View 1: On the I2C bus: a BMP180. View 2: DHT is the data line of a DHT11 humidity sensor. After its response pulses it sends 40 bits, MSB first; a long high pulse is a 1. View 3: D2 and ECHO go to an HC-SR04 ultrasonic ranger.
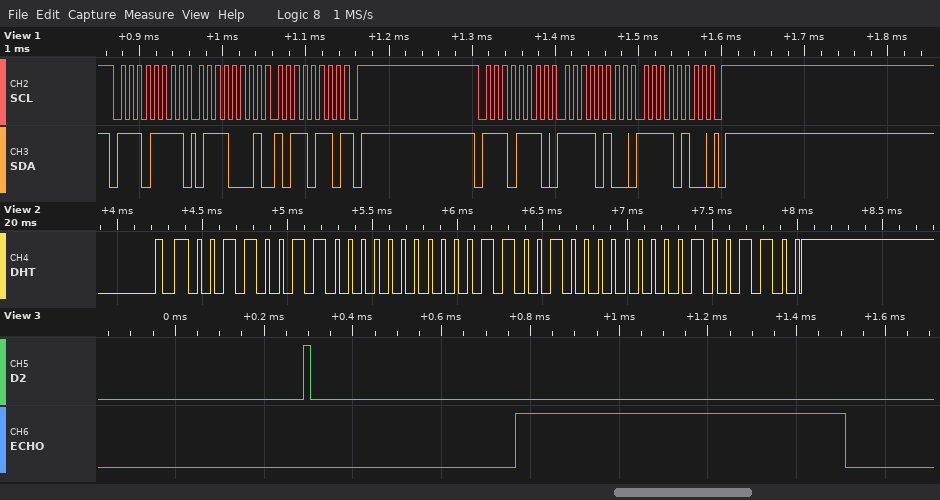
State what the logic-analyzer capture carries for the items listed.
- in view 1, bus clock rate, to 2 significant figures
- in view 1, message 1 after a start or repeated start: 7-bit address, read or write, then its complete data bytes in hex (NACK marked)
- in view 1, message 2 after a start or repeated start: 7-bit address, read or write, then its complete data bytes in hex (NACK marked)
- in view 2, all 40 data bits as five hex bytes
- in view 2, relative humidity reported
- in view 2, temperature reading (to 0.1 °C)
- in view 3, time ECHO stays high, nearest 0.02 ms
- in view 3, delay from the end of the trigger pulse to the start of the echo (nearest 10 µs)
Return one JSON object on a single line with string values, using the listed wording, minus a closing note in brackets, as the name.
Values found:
{"in view 1, bus clock rate, to 2 significant figures": "100 kHz", "in view 1, message 1 after a start or repeated start: 7-bit address, read or write, then its complete data bytes in hex": "0x77 read: 71 B6 NACK", "in view 1, message 2 after a start or repeated start: 7-bit address, read or write, then its complete data bytes in hex": "0x77 write: F4 F4", "in view 2, all 40 data bits as five hex bytes": "33 00 19 00 4C", "in view 2, relative humidity reported": "51 %", "in view 2, temperature reading": "25.0 °C", "in view 3, time ECHO stays high, nearest 0.02 ms": "0.74 ms", "in view 3, delay from the end of the trigger pulse to the start of the echo": "460 µs"}
